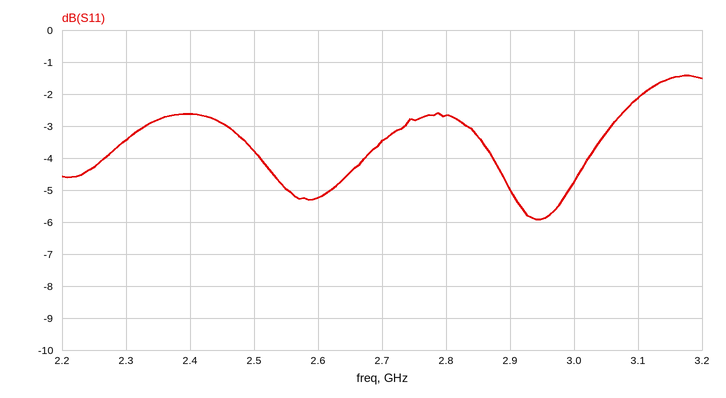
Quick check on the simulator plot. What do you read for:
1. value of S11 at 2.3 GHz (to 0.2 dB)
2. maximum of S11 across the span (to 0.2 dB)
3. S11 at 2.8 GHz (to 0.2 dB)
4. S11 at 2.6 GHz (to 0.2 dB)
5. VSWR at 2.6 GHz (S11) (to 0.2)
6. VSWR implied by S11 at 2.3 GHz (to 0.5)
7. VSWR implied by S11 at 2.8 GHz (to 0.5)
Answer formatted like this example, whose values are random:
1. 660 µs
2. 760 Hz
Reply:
1. -3.4 dB
2. -1.4 dB
3. -2.6 dB
4. -5.2 dB
5. 3.4
6. 5.0
7. 6.5
